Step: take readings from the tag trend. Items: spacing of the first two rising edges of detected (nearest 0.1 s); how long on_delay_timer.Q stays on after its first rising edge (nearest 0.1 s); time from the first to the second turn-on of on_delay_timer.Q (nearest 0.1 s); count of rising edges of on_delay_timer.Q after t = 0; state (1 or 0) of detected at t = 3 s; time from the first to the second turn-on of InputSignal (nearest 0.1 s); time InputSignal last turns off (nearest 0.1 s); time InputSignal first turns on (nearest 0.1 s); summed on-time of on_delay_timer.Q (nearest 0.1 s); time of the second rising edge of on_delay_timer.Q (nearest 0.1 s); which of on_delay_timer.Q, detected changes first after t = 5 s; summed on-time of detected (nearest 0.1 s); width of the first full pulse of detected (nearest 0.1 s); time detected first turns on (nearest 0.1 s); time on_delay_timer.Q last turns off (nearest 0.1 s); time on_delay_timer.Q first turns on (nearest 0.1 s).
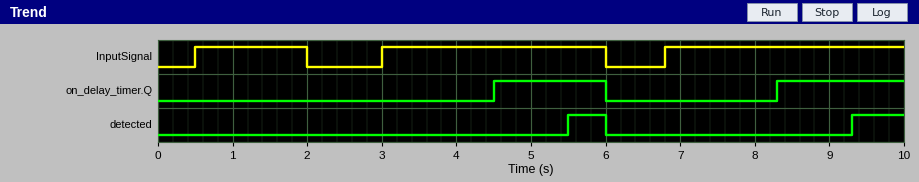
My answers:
3.8 s
1.5 s
3.8 s
2
0
2.5 s
6.0 s
0.5 s
3.2 s
8.3 s
detected
1.2 s
0.5 s
5.5 s
6.0 s
4.5 s
